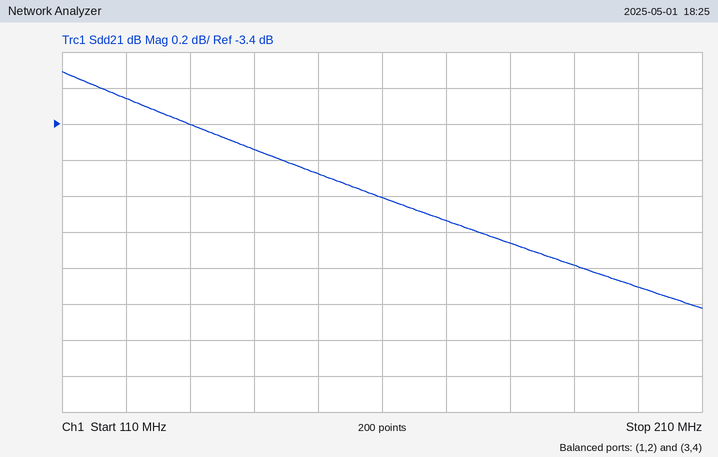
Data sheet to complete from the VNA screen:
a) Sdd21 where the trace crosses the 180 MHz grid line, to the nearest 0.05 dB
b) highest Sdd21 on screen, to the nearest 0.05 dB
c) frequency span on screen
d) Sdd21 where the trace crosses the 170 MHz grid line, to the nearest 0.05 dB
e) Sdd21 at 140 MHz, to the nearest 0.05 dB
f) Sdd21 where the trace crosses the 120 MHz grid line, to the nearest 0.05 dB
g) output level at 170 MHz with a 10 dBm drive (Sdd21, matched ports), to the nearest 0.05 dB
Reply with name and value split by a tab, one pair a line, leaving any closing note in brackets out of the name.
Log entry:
Sdd21 where the trace crosses the 180 MHz grid line, to the nearest 0.05 dB	-4.05 dB
highest Sdd21 on screen, to the nearest 0.05 dB	-3.10 dB
frequency span on screen	100 MHz
Sdd21 where the trace crosses the 170 MHz grid line, to the nearest 0.05 dB	-3.95 dB
Sdd21 at 140 MHz, to the nearest 0.05 dB	-3.55 dB
Sdd21 where the trace crosses the 120 MHz grid line, to the nearest 0.05 dB	-3.25 dB
output level at 170 MHz with a 10 dBm drive (Sdd21, matched ports), to the nearest 0.05 dB	6.05 dBm
